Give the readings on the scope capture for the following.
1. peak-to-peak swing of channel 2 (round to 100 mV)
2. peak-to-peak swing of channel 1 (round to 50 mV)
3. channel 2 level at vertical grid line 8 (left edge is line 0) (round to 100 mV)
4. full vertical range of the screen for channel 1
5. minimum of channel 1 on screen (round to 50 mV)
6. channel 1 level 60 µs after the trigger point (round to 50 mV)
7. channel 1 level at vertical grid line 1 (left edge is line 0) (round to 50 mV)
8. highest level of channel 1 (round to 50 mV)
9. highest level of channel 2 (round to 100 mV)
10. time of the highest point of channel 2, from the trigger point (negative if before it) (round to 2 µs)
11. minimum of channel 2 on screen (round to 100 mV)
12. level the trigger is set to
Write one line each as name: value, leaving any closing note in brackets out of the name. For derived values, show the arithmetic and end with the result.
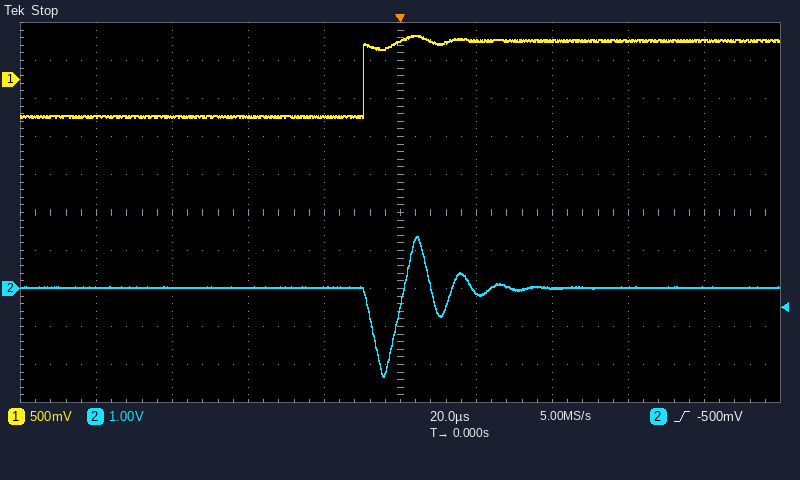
peak-to-peak swing of channel 2: 1.4 V − (-2.3 V) = 3.7 V
peak-to-peak swing of channel 1: 600 mV − (-500 mV) = 1.10 V
channel 2 level at vertical grid line 8 (left edge is line 0): 0.0 V
full vertical range of the screen for channel 1: 5 V
minimum of channel 1 on screen: -500 mV
channel 1 level 60 µs after the trigger point: 500 mV
channel 1 level at vertical grid line 1 (left edge is line 0): -500 mV
highest level of channel 1: 600 mV
highest level of channel 2: 1.4 V
time of the highest point of channel 2, from the trigger point (negative if before it): +4 µs
minimum of channel 2 on screen: -2.3 V
level the trigger is set to: -500 mV
